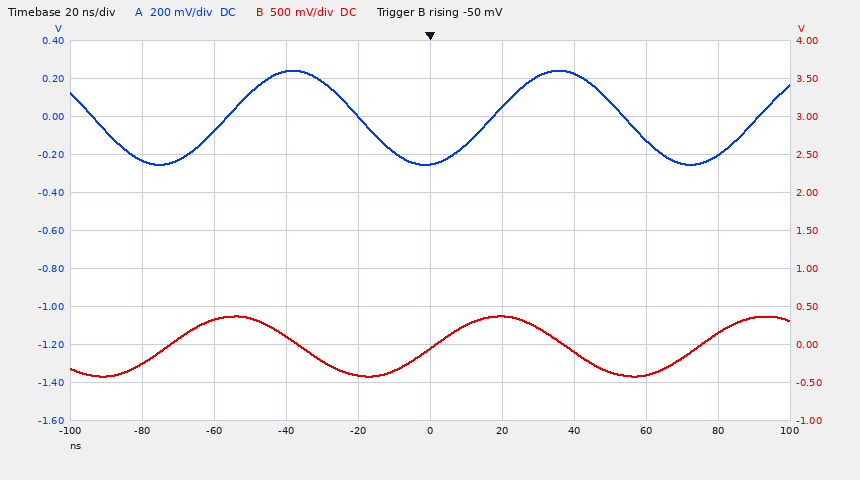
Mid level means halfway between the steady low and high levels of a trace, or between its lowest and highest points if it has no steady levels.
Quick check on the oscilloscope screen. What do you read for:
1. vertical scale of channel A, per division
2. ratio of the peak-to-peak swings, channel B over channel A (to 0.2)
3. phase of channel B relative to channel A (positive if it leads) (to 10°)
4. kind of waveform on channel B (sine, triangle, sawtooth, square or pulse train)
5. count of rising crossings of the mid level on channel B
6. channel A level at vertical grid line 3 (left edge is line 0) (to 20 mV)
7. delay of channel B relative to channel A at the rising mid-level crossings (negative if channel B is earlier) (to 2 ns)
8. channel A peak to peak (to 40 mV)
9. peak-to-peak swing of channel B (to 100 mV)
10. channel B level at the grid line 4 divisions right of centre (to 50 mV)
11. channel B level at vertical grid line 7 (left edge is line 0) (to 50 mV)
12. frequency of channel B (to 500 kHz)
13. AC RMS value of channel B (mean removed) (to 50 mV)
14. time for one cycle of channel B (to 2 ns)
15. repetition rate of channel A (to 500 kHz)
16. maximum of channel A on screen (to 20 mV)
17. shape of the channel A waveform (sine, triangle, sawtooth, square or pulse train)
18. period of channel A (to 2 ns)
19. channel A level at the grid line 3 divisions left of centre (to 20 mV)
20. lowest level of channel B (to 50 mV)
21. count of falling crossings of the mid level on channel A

200 mV
1.6
+80°
sine
3
240 mV
-16 ns
480 mV
800 mV
150 mV
-100 mV
13.5 MHz
300 mV
74 ns
13.5 MHz
240 mV
sine
74 ns
-80 mV
-400 mV
3
